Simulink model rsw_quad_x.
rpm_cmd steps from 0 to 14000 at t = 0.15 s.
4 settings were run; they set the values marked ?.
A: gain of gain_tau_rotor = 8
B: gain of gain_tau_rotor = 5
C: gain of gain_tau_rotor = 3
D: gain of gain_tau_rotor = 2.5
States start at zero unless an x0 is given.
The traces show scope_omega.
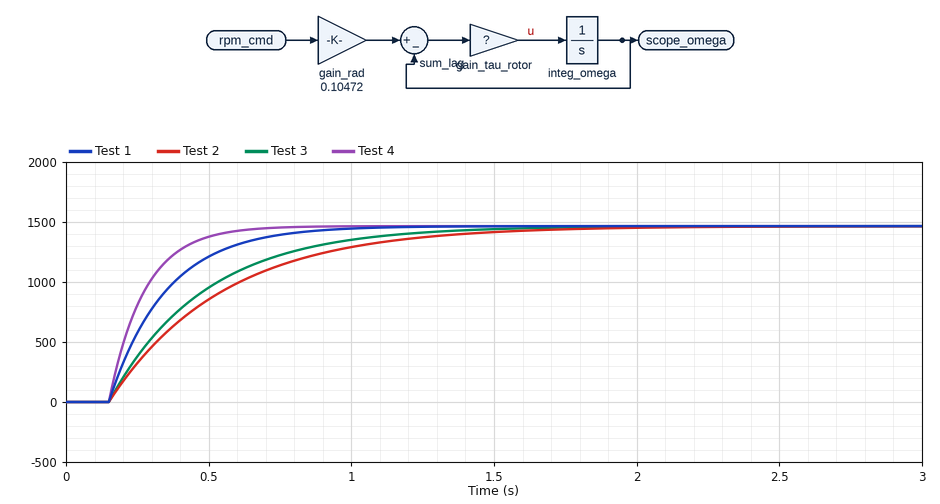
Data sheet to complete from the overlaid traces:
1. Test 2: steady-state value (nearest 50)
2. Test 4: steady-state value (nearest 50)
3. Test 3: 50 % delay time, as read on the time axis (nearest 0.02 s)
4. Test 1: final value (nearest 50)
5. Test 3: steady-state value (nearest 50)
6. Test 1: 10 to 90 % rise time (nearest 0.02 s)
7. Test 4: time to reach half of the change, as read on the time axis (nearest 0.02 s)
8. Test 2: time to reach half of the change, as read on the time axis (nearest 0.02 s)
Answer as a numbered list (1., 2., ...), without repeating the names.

1. 1450
2. 1450
3. 0.38 s
4. 1450
5. 1450
6. 0.44 s
7. 0.24 s
8. 0.42 s
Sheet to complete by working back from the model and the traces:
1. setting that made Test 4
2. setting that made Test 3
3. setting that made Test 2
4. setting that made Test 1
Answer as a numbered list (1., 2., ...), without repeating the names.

1. A
2. C
3. D
4. B
